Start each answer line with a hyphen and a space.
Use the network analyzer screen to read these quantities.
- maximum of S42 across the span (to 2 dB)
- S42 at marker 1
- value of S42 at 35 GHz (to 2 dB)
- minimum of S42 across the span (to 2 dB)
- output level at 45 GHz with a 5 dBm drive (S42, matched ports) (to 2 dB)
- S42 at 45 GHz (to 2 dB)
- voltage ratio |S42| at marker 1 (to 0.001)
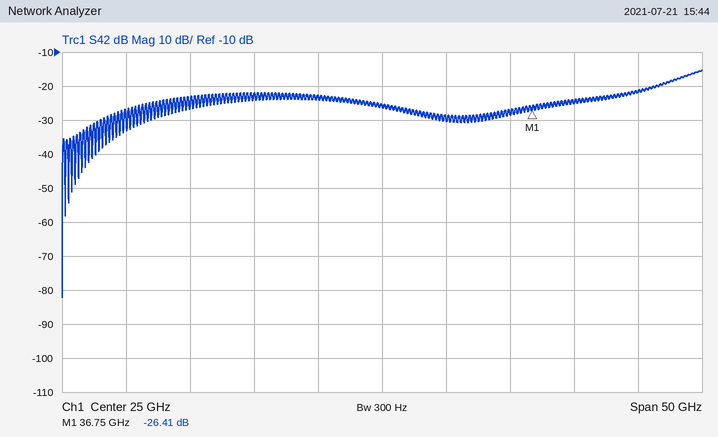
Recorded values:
- -16 dB
- -26.41 dB
- -28 dB
- -82 dB
- -16 dBm
- -22 dB
- 0.048
